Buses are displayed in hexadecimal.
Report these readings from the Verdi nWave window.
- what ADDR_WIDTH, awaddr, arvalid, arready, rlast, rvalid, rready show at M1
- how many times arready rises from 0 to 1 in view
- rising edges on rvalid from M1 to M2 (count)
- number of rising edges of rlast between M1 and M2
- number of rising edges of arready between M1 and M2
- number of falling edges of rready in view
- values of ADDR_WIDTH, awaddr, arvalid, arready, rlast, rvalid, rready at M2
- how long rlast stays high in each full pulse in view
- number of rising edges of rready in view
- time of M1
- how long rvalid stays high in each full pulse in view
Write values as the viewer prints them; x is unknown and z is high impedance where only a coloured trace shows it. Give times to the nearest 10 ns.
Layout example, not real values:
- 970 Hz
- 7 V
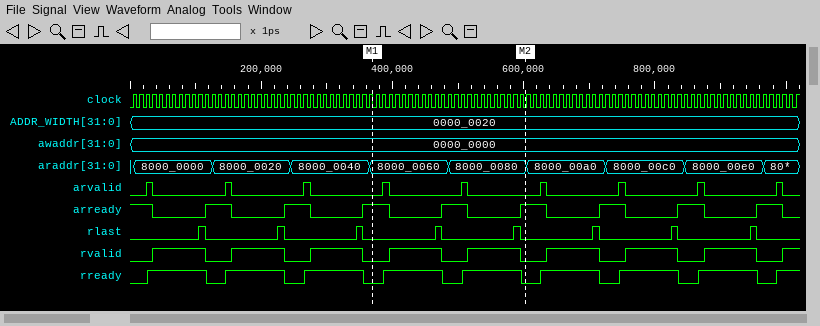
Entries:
- ADDR_WIDTH=0000_0020, awaddr=0000_0000, arvalid=0, arready=1, rlast=0, rvalid=0, rready=0
- 8
- 2
- 2
- 2
- 8
- ADDR_WIDTH=0000_0020, awaddr=0000_0000, arvalid=0, arready=1, rlast=0, rvalid=0, rready=0
- 10 ns, 10 ns, 10 ns, 10 ns, 10 ns, 10 ns, 10 ns, 10 ns
- 9
- 370 ns
- 80 ns, 80 ns, 80 ns, 80 ns, 80 ns, 80 ns, 80 ns, 80 ns
